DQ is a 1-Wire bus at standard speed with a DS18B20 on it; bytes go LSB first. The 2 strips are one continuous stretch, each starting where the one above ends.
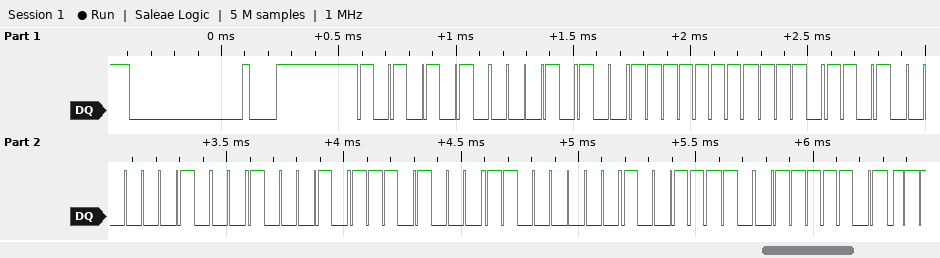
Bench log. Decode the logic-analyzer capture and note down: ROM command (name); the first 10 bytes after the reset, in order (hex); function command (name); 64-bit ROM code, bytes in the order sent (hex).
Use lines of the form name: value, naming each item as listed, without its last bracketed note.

ROM command: Match ROM
the first 10 bytes after the reset, in order: 55 28 FF B7 40 44 17 03 79 BE
function command: Read Scratchpad
64-bit ROM code, bytes in the order sent: 28 FF B7 40 44 17 03 79
